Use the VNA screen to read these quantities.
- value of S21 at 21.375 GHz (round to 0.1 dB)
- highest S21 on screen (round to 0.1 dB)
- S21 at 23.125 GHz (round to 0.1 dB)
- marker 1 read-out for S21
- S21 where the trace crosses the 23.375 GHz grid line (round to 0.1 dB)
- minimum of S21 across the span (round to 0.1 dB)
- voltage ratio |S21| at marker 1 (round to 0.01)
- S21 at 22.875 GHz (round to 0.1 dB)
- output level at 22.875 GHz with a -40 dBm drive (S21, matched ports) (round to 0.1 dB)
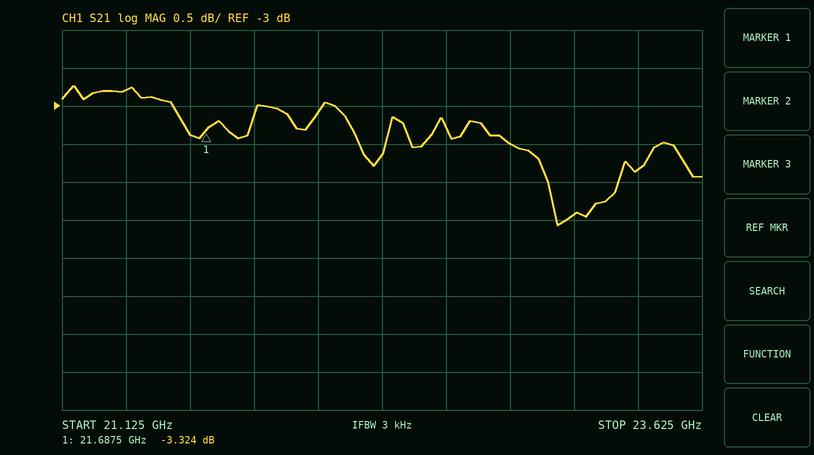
-2.8 dB
-2.7 dB
-4.4 dB
-3.324 dB
-3.8 dB
-4.6 dB
0.68
-3.5 dB
-43.5 dBm
